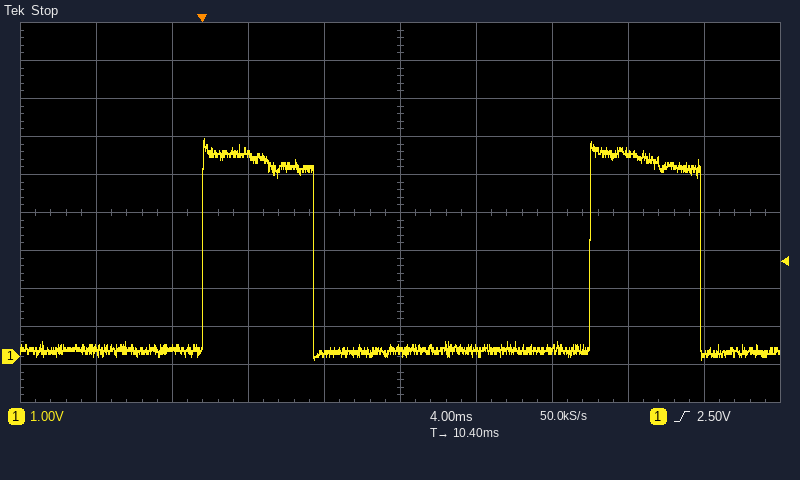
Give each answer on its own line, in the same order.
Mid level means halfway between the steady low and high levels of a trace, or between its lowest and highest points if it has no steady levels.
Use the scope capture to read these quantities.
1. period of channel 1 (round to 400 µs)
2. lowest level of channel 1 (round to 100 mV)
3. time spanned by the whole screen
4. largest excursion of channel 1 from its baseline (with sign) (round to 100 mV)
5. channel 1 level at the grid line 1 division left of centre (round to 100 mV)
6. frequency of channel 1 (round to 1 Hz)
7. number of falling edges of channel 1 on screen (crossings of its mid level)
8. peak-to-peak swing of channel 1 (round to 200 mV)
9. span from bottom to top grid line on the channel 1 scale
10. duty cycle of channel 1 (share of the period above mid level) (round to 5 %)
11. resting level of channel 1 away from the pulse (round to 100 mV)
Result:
20.4 ms
-100 mV
40 ms
+5.6 V
100 mV
49 Hz
2
5.8 V
10 V
30 %
200 mV
